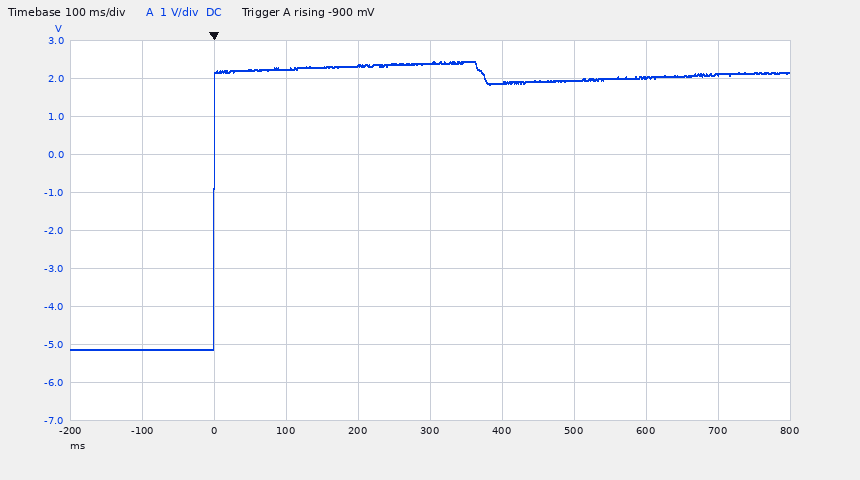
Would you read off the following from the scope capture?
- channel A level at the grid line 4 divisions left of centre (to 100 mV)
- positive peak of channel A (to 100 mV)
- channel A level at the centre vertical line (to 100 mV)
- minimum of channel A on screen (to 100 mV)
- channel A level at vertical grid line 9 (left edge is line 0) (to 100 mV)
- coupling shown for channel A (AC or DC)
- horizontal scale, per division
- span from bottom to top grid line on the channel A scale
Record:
-5.1 V
2.4 V
2.4 V
-5.1 V
2.1 V
DC
100 ms
10 V
